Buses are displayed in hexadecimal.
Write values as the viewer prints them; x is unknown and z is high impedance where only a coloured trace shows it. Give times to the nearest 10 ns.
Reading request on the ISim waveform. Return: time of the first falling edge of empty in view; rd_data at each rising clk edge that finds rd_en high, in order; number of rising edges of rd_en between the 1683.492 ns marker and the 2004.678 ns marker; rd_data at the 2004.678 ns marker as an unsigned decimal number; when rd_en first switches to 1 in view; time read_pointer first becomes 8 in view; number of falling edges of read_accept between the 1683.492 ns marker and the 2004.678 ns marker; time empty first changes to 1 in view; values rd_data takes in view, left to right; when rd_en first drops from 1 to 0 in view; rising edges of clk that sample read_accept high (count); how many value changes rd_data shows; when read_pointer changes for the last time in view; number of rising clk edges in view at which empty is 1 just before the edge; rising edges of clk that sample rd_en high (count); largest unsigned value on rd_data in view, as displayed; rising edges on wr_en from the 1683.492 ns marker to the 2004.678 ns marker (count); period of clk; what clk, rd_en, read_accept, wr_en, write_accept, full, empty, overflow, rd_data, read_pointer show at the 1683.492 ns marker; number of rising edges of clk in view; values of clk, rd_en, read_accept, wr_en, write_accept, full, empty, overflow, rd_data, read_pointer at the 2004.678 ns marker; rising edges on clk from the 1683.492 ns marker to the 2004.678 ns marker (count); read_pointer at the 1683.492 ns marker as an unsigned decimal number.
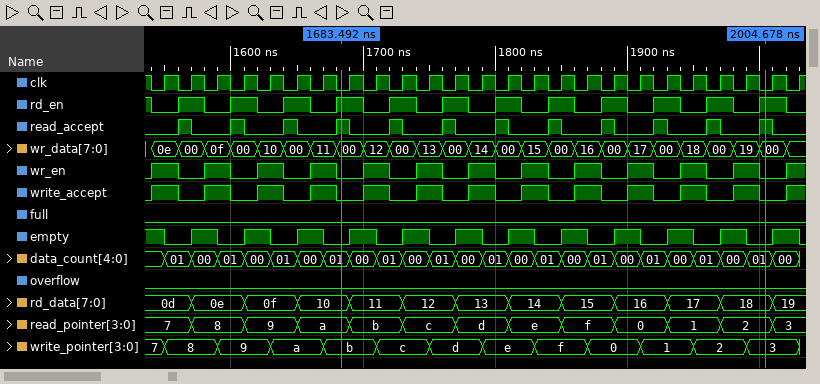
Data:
1550 ns
0d, 0e, 0f, 10, 11, 12, 13, 14, 15, 16, 17, 18
8
24
1560 ns
1570 ns
8
1570 ns
0d, 0e, 0f, 10, 11, 12, 13, 14, 15, 16, 17, 18, 19
1540 ns
12
12
2010 ns
13
12
19
8
20 ns
clk=0, rd_en=1, read_accept=1, wr_en=0, write_accept=0, full=0, empty=0, overflow=0, rd_data=10, read_pointer=a
25
clk=0, rd_en=1, read_accept=1, wr_en=0, write_accept=0, full=0, empty=0, overflow=0, rd_data=18, read_pointer=2
16
10
